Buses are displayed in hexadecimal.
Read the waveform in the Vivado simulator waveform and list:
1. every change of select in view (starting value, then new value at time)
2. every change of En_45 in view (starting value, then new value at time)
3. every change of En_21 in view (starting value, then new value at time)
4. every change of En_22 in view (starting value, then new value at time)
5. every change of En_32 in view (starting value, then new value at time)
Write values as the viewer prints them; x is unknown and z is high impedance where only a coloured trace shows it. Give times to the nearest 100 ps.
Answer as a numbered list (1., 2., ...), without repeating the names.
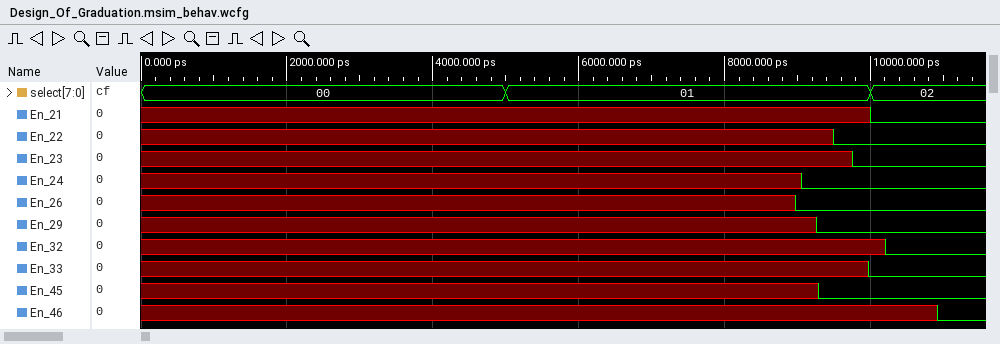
1. 00, 01 at 5000 ps, 02 at 10000 ps
2. x, 0 at 9300 ps
3. x, 0 at 10000 ps
4. x, 0 at 9500 ps
5. x, 0 at 10200 ps
